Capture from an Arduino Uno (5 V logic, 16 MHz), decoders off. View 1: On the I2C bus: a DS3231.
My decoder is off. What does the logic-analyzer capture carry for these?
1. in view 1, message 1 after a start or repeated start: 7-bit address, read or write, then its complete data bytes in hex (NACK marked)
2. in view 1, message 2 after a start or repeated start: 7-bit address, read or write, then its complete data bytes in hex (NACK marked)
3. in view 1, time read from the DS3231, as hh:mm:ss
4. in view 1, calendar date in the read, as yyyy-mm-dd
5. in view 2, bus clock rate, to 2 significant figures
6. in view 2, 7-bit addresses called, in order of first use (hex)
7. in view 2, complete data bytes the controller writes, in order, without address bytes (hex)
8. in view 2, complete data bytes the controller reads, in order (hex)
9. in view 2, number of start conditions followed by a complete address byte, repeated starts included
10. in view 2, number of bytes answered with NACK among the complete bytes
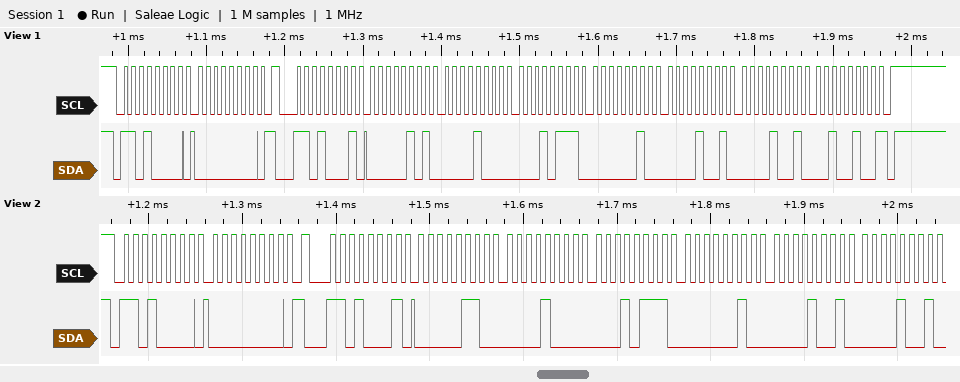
0x68 write: 00
0x68 read: 05 08 17 02 09 09 24 NACK
17:08:05
2024-09-09
100 kHz
0x68
00
06 08 17 02 09 09
2
0
